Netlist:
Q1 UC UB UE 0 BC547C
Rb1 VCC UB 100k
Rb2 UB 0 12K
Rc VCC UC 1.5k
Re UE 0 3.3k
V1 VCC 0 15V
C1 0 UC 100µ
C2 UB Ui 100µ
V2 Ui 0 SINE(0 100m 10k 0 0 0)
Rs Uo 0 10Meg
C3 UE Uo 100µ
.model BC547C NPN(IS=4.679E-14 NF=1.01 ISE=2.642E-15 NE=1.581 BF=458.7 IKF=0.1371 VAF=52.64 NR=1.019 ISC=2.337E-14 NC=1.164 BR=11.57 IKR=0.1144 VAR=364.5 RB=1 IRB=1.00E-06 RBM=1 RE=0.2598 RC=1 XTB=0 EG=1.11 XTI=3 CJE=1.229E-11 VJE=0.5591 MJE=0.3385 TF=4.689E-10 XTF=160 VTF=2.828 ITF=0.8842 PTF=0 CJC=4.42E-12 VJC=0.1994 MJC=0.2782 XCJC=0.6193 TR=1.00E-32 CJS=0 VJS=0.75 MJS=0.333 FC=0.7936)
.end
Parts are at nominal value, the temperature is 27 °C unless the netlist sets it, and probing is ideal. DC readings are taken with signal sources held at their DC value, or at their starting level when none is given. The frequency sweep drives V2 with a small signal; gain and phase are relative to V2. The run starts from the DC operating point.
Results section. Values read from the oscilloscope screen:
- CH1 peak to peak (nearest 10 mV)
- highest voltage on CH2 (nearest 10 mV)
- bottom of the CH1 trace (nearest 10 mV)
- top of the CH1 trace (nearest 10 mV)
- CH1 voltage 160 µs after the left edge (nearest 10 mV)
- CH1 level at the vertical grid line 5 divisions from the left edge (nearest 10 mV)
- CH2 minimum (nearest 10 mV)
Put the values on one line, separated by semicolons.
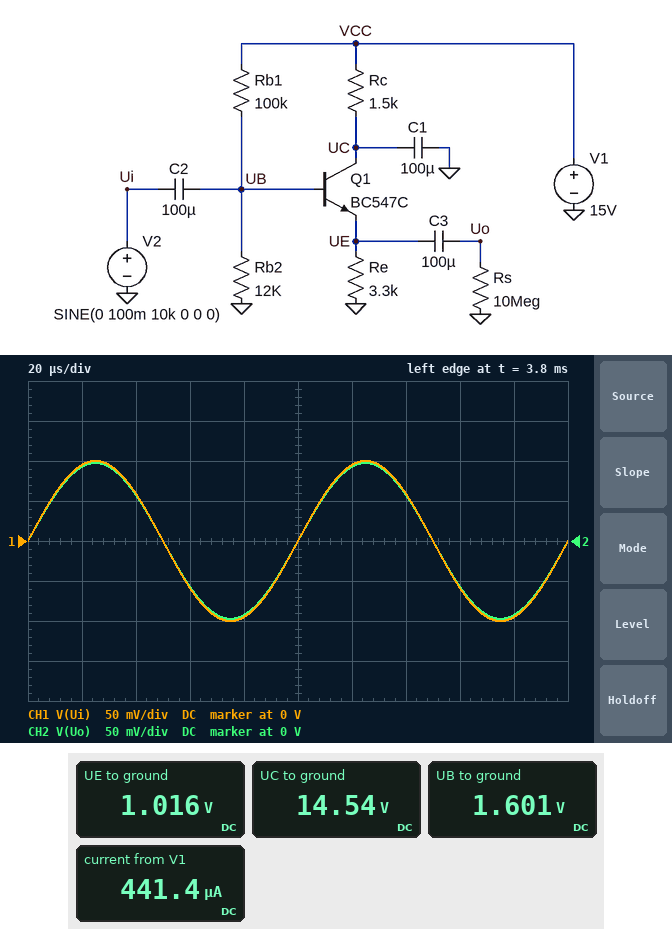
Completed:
200 mV; 100 mV; -100 mV; 100 mV; -60 mV; 0 V; -100 mV
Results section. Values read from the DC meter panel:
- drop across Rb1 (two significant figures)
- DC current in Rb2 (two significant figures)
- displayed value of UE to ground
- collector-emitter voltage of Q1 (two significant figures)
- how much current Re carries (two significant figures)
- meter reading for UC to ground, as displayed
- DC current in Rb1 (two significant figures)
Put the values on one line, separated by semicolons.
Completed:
13 V; 130 µA; 1.016 V; 14 V; 310 µA; 14.54 V; 130 µA
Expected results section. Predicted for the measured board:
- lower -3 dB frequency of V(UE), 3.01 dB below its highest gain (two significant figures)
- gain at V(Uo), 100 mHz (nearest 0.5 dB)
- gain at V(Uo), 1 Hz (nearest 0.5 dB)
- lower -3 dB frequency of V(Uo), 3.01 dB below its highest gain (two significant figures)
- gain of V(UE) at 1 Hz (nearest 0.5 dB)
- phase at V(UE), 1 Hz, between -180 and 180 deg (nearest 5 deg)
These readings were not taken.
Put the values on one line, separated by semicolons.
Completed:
150 mHz; -5.5 dB; -0.5 dB; 150 mHz; -0.5 dB; 10 deg
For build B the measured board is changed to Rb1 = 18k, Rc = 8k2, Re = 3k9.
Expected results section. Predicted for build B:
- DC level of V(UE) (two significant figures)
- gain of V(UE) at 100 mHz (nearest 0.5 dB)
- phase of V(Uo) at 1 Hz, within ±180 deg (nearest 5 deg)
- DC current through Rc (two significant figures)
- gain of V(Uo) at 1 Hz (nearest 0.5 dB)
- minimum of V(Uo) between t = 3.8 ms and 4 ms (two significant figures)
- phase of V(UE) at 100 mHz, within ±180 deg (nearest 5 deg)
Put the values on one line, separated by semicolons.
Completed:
5.0 V; -18.5 dB; 25 deg; 1.2 mA; -6.5 dB; -100 mV; 75 deg
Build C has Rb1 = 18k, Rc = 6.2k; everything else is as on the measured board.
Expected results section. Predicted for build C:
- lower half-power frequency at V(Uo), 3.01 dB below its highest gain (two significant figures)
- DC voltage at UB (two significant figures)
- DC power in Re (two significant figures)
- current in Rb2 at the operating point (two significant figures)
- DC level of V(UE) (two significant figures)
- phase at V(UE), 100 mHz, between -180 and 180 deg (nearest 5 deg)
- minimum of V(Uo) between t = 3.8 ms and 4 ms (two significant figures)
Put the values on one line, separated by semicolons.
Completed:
1.1 Hz; 5.9 V; 8.3 mW; 490 µA; 5.2 V; 80 deg; -100 mV
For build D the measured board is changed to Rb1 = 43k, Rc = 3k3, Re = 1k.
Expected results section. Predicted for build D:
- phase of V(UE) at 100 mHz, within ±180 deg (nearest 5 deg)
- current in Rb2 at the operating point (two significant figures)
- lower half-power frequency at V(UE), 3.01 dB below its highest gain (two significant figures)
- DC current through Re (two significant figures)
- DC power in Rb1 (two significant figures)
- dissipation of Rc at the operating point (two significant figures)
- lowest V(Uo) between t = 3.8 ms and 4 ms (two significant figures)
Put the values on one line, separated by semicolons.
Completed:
60 deg; 270 µA; 170 mHz; 2.6 mA; 3.2 mW; 22 mW; -99 mV
